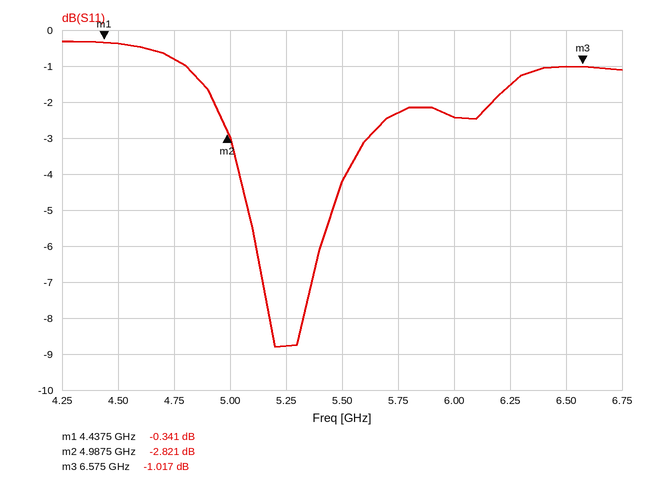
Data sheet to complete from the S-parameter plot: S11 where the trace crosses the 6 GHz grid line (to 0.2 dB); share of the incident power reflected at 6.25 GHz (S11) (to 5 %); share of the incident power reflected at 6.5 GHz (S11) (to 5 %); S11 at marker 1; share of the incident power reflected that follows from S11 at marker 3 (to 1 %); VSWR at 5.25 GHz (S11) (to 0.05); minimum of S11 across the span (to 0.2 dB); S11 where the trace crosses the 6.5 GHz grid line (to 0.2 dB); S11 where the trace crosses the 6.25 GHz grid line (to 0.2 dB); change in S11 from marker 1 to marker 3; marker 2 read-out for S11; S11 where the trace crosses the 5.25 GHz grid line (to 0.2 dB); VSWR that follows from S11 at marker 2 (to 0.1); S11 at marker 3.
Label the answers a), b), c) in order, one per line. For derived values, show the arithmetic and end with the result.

a) -2.4 dB
b) 10^(-1.6/10) ≈ 69.2 %, so 70 % to the nearest 5 %
c) 10^(-1/10) ≈ 79.4 %, so 80 % to the nearest 5 %
d) -0.341 dB
e) 10^(-1.017/10) ≈ 79 %
f) |Γ| = 10^(-8.8/20) = 0.3631; VSWR = (1 + 0.3631)/(1 − 0.3631) ≈ 2.14, so 2.15 to the nearest 0.05
g) -8.8 dB
h) -1.0 dB
i) -1.6 dB
j) -1.017 − (-0.341) = -0.676 dB
k) -2.821 dB
l) -8.8 dB
m) (1 + 0.7227)/(1 − 0.7227) ≈ 6.2
n) -1.017 dB
